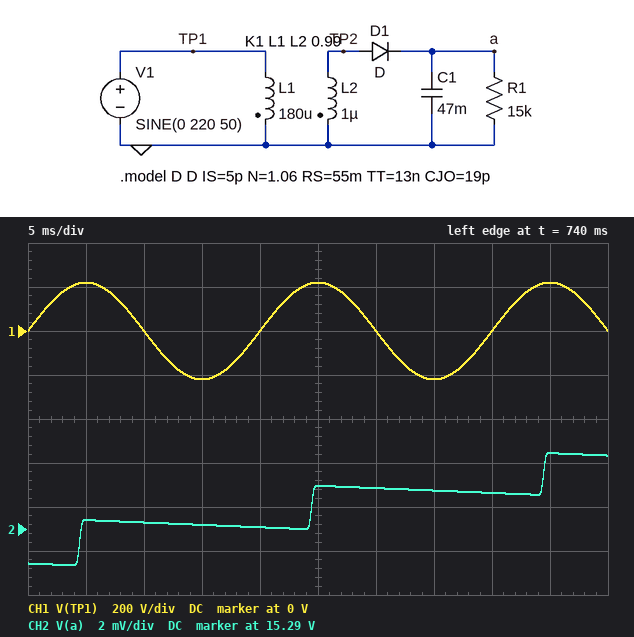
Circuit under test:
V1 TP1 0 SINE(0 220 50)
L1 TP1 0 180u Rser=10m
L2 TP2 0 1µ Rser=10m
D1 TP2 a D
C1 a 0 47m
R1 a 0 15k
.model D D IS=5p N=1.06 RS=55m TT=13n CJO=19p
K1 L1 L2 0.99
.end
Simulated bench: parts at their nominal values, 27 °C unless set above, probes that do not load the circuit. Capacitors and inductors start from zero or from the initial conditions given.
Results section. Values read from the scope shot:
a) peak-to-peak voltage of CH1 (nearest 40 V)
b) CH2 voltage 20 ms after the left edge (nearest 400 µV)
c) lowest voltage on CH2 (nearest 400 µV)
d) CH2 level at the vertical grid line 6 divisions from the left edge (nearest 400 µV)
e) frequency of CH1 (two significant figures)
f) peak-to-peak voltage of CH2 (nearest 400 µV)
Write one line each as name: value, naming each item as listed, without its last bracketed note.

peak-to-peak voltage of CH1: 440 V
CH2 voltage 20 ms after the left edge: 15.2940 V
lowest voltage on CH2: 15.2924 V
CH2 level at the vertical grid line 6 divisions from the left edge: 15.2960 V
frequency of CH1: 50 Hz
peak-to-peak voltage of CH2: 5.2 mV
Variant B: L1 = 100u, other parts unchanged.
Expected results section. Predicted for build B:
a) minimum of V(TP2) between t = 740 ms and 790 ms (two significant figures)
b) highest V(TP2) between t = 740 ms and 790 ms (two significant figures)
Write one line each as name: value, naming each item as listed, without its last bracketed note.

minimum of V(TP2) between t = 740 ms and 790 ms: -21 V
highest V(TP2) between t = 740 ms and 790 ms: 21 V
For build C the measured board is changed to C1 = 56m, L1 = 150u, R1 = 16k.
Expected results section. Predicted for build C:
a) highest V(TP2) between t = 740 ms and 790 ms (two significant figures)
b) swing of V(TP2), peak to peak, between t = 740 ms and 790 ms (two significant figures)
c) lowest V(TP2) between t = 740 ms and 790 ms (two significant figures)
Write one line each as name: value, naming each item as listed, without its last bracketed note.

highest V(TP2) between t = 740 ms and 790 ms: 17 V
swing of V(TP2), peak to peak, between t = 740 ms and 790 ms: 35 V
lowest V(TP2) between t = 740 ms and 790 ms: -17 V
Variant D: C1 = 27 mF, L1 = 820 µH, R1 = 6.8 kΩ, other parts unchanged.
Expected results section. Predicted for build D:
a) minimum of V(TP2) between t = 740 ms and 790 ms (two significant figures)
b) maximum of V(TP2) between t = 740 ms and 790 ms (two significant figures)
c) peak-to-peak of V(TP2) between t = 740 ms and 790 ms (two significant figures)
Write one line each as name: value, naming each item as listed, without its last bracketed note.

minimum of V(TP2) between t = 740 ms and 790 ms: -7.6 V
maximum of V(TP2) between t = 740 ms and 790 ms: 7.6 V
peak-to-peak of V(TP2) between t = 740 ms and 790 ms: 15 V
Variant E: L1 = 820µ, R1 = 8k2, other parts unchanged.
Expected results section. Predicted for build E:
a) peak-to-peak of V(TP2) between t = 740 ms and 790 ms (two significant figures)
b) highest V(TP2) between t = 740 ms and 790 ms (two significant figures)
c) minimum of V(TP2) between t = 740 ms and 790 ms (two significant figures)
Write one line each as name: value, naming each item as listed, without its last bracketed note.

peak-to-peak of V(TP2) between t = 740 ms and 790 ms: 15 V
highest V(TP2) between t = 740 ms and 790 ms: 7.6 V
minimum of V(TP2) between t = 740 ms and 790 ms: -7.6 V
